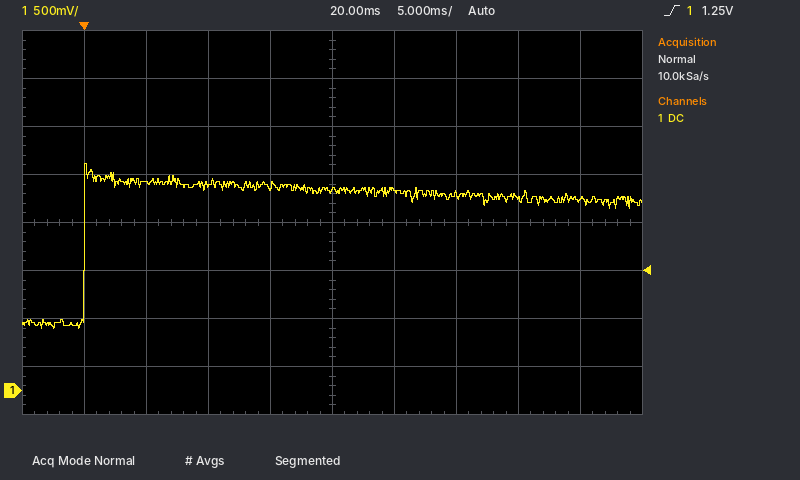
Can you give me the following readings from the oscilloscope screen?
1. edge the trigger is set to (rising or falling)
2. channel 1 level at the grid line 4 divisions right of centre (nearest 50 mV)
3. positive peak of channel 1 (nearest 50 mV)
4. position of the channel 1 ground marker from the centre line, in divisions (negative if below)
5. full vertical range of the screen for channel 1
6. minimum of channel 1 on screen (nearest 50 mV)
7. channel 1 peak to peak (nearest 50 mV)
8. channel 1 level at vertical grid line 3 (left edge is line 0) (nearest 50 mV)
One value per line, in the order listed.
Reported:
rising
2.00 V
2.35 V
-3.5 div
4 V
650 mV
1.70 V
2.15 V
